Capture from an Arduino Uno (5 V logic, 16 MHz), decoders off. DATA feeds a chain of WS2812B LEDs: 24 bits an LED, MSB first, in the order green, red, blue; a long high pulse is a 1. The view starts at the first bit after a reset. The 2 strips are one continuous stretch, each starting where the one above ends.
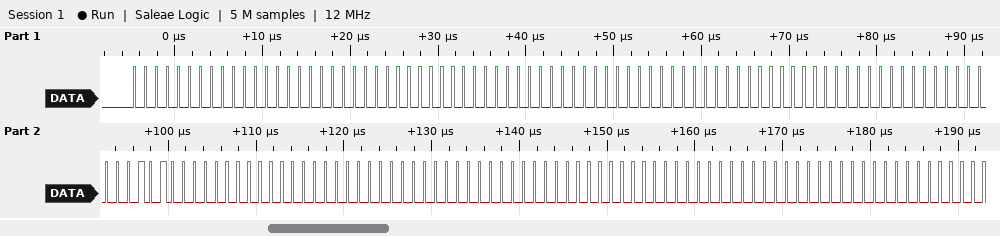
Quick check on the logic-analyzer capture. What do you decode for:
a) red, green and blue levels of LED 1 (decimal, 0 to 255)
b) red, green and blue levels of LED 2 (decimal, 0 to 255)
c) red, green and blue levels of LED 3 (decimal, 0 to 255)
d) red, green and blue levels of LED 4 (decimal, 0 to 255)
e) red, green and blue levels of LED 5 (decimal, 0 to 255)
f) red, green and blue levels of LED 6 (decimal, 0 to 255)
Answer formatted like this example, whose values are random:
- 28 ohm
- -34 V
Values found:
- 0, 0, 0
- 0, 0, 0
- 0, 0, 0
- 80, 0, 0
- 0, 0, 0
- 0, 0, 0
